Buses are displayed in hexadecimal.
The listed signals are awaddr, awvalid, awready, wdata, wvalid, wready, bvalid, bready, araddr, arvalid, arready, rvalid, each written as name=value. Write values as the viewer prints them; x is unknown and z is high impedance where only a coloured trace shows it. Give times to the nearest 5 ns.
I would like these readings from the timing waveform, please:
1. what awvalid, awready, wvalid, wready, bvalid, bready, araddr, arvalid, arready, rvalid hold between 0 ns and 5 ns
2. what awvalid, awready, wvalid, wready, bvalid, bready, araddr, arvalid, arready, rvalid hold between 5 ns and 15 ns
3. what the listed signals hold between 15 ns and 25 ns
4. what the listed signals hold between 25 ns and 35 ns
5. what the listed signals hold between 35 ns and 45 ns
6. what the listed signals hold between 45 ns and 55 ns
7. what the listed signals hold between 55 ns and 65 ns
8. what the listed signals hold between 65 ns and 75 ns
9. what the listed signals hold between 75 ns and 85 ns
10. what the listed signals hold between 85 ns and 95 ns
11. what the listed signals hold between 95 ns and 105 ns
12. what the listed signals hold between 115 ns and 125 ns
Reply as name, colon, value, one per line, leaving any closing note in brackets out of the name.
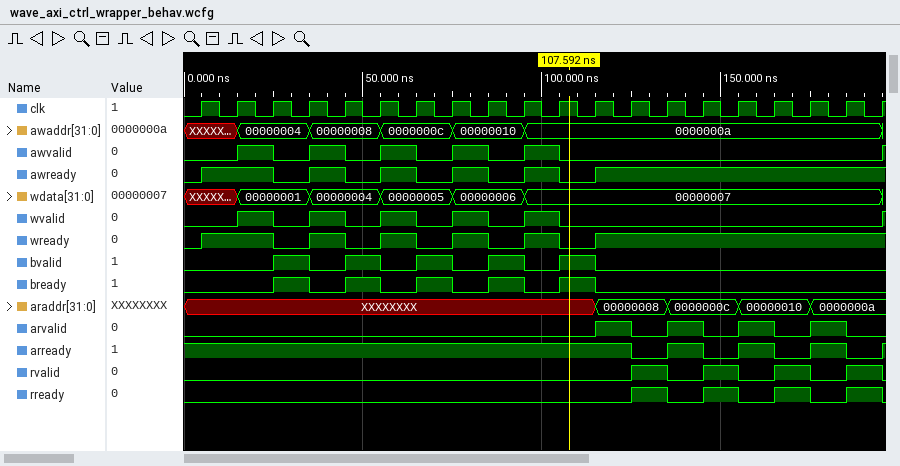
what awvalid, awready, wvalid, wready, bvalid, bready, araddr, arvalid, arready, rvalid hold between 0 ns and 5 ns: awvalid=0, awready=0, wvalid=0, wready=0, bvalid=0, bready=0, araddr=XXXXXXXX, arvalid=0, arready=1, rvalid=0
what awvalid, awready, wvalid, wready, bvalid, bready, araddr, arvalid, arready, rvalid hold between 5 ns and 15 ns: awvalid=0, awready=1, wvalid=0, wready=1, bvalid=0, bready=0, araddr=XXXXXXXX, arvalid=0, arready=1, rvalid=0
what the listed signals hold between 15 ns and 25 ns: awaddr=00000004, awvalid=1, awready=1, wdata=00000001, wvalid=1, wready=1, bvalid=0, bready=0, araddr=XXXXXXXX, arvalid=0, arready=1, rvalid=0
what the listed signals hold between 25 ns and 35 ns: awaddr=00000004, awvalid=0, awready=0, wdata=00000001, wvalid=0, wready=0, bvalid=1, bready=1, araddr=XXXXXXXX, arvalid=0, arready=1, rvalid=0
what the listed signals hold between 35 ns and 45 ns: awaddr=00000008, awvalid=1, awready=1, wdata=00000004, wvalid=1, wready=1, bvalid=0, bready=0, araddr=XXXXXXXX, arvalid=0, arready=1, rvalid=0
what the listed signals hold between 45 ns and 55 ns: awaddr=00000008, awvalid=0, awready=0, wdata=00000004, wvalid=0, wready=0, bvalid=1, bready=1, araddr=XXXXXXXX, arvalid=0, arready=1, rvalid=0
what the listed signals hold between 55 ns and 65 ns: awaddr=0000000c, awvalid=1, awready=1, wdata=00000005, wvalid=1, wready=1, bvalid=0, bready=0, araddr=XXXXXXXX, arvalid=0, arready=1, rvalid=0
what the listed signals hold between 65 ns and 75 ns: awaddr=0000000c, awvalid=0, awready=0, wdata=00000005, wvalid=0, wready=0, bvalid=1, bready=1, araddr=XXXXXXXX, arvalid=0, arready=1, rvalid=0
what the listed signals hold between 75 ns and 85 ns: awaddr=00000010, awvalid=1, awready=1, wdata=00000006, wvalid=1, wready=1, bvalid=0, bready=0, araddr=XXXXXXXX, arvalid=0, arready=1, rvalid=0
what the listed signals hold between 85 ns and 95 ns: awaddr=00000010, awvalid=0, awready=0, wdata=00000006, wvalid=0, wready=0, bvalid=1, bready=1, araddr=XXXXXXXX, arvalid=0, arready=1, rvalid=0
what the listed signals hold between 95 ns and 105 ns: awaddr=0000000a, awvalid=1, awready=1, wdata=00000007, wvalid=1, wready=1, bvalid=0, bready=0, araddr=XXXXXXXX, arvalid=0, arready=1, rvalid=0
what the listed signals hold between 115 ns and 125 ns: awaddr=0000000a, awvalid=0, awready=1, wdata=00000007, wvalid=0, wready=1, bvalid=0, bready=0, araddr=00000008, arvalid=1, arready=1, rvalid=0
